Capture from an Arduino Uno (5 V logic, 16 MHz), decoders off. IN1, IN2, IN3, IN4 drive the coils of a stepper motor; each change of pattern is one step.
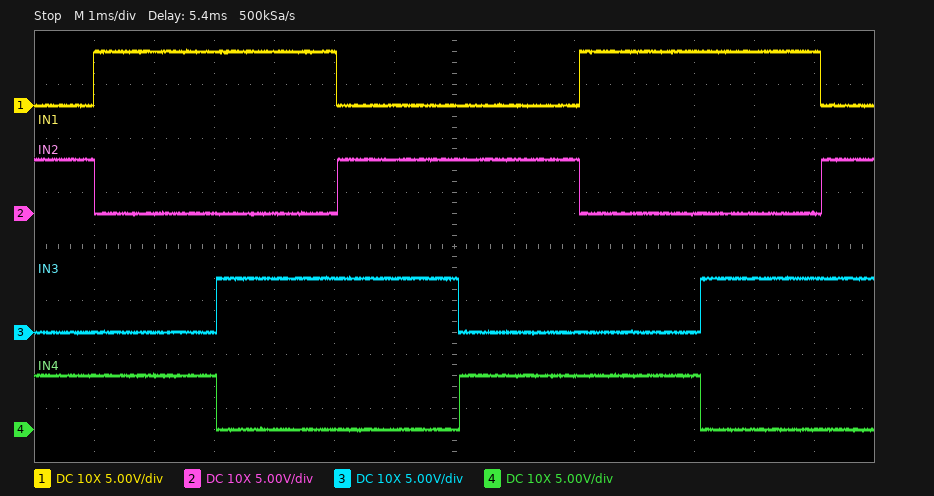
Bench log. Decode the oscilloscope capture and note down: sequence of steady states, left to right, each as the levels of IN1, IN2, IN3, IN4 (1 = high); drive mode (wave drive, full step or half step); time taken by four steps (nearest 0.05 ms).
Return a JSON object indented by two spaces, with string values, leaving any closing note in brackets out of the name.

{
  "sequence of steady states, left to right, each as the levels of IN1, IN2, IN3, IN4": "0101 1001 1010 0110 0101 1001 1010 0110",
  "drive mode": "full step",
  "time taken by four steps": "8.10 ms"
}
